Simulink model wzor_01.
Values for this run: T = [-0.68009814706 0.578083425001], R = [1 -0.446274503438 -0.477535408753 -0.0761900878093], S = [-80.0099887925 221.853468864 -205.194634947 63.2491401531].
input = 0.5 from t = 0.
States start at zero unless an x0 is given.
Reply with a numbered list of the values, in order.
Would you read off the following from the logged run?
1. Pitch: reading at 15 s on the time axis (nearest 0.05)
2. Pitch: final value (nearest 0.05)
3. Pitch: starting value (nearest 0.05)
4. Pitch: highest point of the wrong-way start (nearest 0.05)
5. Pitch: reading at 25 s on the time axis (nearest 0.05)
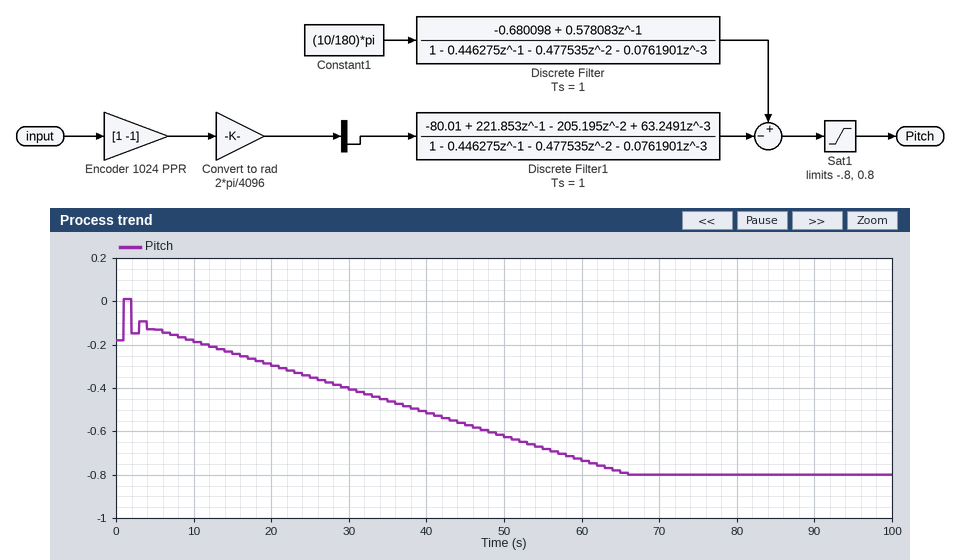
1. -0.25
2. -0.80
3. -0.20
4. 0.00
5. -0.35
